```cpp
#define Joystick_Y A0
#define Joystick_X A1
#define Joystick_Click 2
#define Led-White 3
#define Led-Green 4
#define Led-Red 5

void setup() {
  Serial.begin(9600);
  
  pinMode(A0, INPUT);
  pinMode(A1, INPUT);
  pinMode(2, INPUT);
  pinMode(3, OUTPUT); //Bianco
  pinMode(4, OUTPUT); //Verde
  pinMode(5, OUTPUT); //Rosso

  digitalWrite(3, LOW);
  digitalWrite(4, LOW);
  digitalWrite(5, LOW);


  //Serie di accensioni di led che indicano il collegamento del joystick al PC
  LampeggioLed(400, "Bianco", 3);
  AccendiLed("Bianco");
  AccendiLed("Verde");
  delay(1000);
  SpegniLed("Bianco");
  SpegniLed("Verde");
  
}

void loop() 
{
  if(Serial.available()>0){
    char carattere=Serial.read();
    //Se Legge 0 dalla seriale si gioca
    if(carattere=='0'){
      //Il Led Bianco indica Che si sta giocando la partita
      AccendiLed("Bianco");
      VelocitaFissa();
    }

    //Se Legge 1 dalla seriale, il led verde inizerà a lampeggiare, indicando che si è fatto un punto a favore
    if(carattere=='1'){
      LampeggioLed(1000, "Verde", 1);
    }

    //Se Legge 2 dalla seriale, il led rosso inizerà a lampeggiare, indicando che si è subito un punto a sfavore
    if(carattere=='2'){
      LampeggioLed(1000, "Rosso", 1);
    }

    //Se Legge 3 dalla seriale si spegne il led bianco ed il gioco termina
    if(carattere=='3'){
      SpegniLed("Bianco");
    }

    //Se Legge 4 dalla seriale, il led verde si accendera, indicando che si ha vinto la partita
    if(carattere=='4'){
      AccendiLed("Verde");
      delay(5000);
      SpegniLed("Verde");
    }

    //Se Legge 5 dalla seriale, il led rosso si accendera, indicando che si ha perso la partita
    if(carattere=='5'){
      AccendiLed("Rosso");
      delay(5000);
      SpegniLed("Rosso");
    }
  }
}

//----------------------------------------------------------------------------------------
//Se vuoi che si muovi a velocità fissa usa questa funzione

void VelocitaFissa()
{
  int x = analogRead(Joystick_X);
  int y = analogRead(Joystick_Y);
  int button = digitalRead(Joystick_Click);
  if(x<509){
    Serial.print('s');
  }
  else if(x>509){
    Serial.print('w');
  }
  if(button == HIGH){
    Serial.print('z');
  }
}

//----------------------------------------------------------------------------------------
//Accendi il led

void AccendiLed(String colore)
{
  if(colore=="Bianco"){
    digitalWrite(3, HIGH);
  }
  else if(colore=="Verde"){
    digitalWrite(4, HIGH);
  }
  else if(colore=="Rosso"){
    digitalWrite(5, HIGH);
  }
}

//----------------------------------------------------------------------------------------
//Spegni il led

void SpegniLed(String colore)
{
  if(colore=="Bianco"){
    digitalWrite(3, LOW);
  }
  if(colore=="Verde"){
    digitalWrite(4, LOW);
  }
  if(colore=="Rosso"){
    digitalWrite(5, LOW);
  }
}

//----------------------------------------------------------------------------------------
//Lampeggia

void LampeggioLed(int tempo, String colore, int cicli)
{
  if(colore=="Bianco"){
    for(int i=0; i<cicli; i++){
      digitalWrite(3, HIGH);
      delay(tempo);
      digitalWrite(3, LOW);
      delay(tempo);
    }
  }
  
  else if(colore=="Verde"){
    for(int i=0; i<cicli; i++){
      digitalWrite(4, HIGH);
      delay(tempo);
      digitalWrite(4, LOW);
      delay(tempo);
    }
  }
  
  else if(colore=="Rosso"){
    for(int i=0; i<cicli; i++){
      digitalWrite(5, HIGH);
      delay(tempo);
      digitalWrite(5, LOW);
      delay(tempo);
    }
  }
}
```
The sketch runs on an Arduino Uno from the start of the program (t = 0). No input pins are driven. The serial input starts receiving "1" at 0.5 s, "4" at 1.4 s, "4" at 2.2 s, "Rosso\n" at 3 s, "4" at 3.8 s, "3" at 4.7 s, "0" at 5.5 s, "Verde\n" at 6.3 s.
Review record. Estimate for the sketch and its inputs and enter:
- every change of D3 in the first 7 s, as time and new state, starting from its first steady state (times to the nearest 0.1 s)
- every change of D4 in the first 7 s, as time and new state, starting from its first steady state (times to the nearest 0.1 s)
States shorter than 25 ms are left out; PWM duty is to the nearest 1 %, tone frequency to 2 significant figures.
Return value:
0 s high; 0.4 s low; 0.8 s high; 1.2 s low; 1.6 s high; 2 s low; 2.4 s high; 3.4 s low
0 s low; 2.4 s high; 4.4 s low; 5.4 s high
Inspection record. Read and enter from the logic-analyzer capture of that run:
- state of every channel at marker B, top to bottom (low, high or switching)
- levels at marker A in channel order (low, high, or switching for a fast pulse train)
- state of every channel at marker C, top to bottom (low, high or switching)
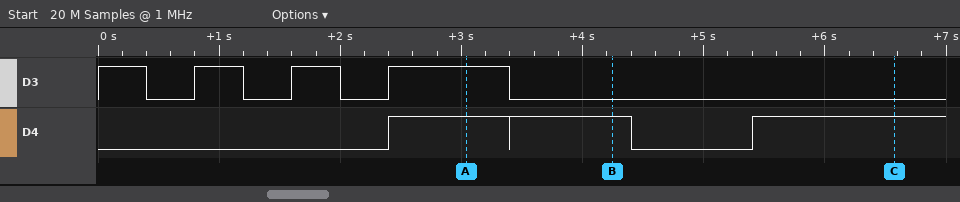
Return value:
D3 low, D4 high
D3 high, D4 high
D3 low, D4 high
